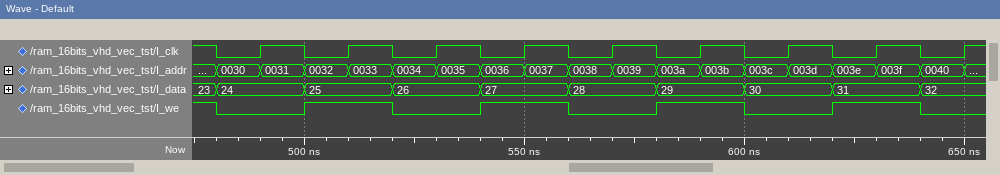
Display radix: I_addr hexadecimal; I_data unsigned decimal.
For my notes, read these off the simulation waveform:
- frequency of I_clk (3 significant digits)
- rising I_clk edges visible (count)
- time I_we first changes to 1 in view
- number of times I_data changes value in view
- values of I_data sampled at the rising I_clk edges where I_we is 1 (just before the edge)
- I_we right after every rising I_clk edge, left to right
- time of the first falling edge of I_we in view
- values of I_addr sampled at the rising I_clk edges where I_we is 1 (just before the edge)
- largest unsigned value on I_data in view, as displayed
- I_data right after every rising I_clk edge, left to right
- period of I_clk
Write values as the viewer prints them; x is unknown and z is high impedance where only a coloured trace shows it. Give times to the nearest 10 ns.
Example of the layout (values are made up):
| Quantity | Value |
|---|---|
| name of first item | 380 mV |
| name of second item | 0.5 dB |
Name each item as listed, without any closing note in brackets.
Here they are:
| Quantity | Value |
|---|---|
| frequency of I_clk | 50.0 MHz |
| rising I_clk edges visible | 9 |
| time I_we first changes to 1 in view | 500 ns |
| number of times I_data changes value in view | 9 |
| values of I_data sampled at the rising I_clk edges where I_we is 1 | 25, 27, 29, 31 |
| I_we right after every rising I_clk edge, left to right | 0 1 0 1 0 1 0 1 0 |
| time of the first falling edge of I_we in view | 480 ns |
| values of I_addr sampled at the rising I_clk edges where I_we is 1 | 0032, 0036, 003a, 003e |
| largest unsigned value on I_data in view, as displayed | 32 |
| I_data right after every rising I_clk edge, left to right | 24, 25, 26, 27, 28, 29, 30, 31, 32 |
| period of I_clk | 20 ns |
